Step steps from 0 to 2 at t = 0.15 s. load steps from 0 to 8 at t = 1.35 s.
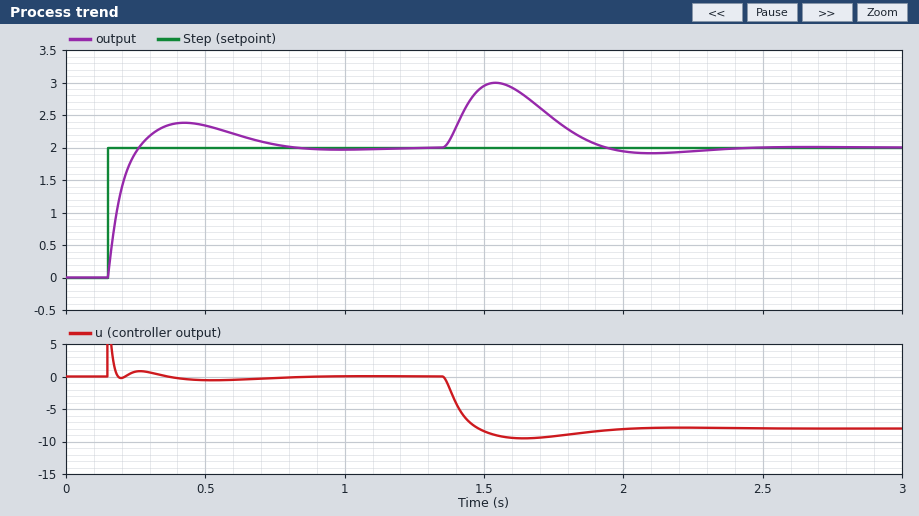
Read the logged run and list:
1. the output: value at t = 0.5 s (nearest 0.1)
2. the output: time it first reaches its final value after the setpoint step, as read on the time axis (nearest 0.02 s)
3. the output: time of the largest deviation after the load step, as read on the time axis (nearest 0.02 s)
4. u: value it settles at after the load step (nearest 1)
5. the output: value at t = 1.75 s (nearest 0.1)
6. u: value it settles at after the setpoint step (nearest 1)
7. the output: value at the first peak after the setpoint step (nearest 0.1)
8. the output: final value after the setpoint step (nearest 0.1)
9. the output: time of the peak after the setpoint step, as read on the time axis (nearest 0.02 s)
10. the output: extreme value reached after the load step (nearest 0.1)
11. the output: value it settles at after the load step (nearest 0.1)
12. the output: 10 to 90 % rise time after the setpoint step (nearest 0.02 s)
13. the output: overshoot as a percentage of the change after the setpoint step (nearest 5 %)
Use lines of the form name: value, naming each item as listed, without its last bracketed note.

the output: value at t = 0.5 s: 2.3
the output: time it first reaches its final value after the setpoint step, as read on the time axis: 0.26 s
the output: time of the largest deviation after the load step, as read on the time axis: 1.54 s
u: value it settles at after the load step: -8
the output: value at t = 1.75 s: 2.4
u: value it settles at after the setpoint step: 0
the output: value at the first peak after the setpoint step: 2.4
the output: final value after the setpoint step: 2.0
the output: time of the peak after the setpoint step, as read on the time axis: 0.42 s
the output: extreme value reached after the load step: 3.0
the output: value it settles at after the load step: 2.0
the output: 10 to 90 % rise time after the setpoint step: 0.08 s
the output: overshoot as a percentage of the change after the setpoint step: 20 %
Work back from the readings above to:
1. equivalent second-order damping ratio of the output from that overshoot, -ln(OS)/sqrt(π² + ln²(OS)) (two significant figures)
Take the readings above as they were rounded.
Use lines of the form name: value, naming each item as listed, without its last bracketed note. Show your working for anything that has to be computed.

equivalent second-order damping ratio of the output from that overshoot, -ln(OS)/sqrt(π² + ln²(OS)): ln(0.2) = -1.609; 1.609 / sqrt(9.870 + 2.590) = 0.46
